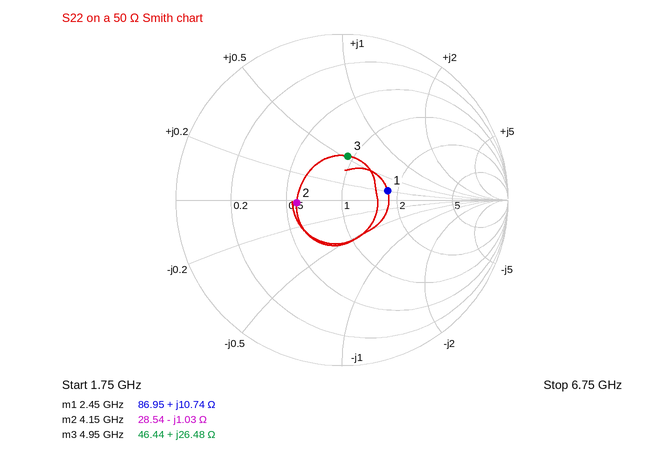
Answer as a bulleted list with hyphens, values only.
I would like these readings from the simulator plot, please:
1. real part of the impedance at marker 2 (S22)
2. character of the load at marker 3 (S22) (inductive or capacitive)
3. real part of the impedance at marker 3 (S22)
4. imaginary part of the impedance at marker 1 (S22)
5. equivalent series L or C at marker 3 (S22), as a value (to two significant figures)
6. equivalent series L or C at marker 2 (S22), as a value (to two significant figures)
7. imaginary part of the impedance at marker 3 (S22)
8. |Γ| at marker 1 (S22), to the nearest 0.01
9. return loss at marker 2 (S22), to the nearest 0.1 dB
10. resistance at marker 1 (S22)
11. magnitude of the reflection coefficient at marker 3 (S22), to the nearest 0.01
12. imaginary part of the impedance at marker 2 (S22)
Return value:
- 28.54 Ω
- inductive
- 46.44 Ω
- +10.74 Ω
- 850 pH
- 37 pF
- +26.48 Ω
- 0.28
- 11.3 dB
- 86.95 Ω
- 0.27
- -1.03 Ω
